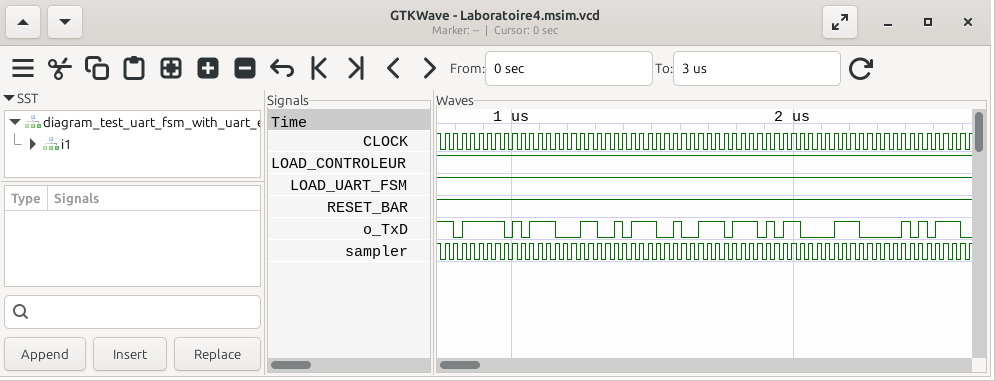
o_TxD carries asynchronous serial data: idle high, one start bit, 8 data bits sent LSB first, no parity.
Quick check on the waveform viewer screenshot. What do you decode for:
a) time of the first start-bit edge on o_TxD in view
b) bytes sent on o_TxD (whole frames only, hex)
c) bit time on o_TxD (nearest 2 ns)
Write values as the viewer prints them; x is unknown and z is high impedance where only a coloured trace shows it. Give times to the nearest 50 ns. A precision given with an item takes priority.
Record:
800 ns
5F, 4C, 72, 0D, 50
30 ns
